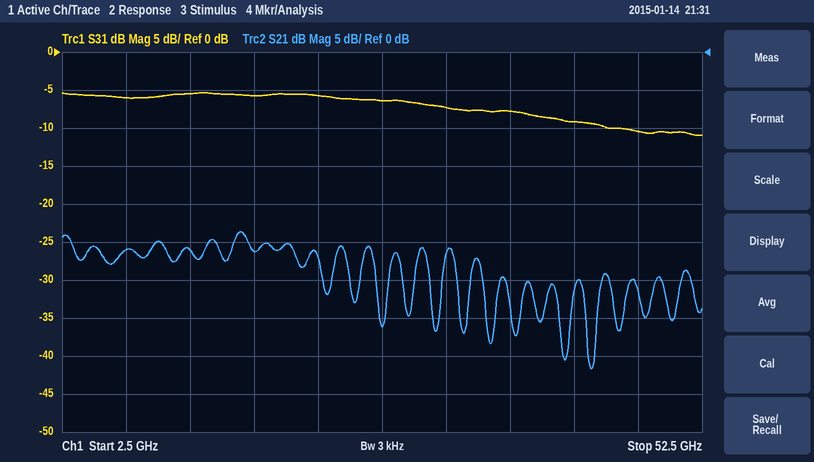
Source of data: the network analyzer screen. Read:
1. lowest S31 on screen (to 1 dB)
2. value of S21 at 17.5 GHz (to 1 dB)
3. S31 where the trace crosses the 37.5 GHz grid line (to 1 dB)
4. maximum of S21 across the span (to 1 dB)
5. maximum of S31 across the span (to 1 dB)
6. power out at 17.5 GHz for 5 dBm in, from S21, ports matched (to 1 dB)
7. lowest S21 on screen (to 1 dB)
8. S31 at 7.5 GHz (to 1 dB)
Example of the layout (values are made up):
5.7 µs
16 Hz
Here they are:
-11 dB
-26 dB
-8 dB
-24 dB
-5 dB
-21 dBm
-42 dB
-6 dB
